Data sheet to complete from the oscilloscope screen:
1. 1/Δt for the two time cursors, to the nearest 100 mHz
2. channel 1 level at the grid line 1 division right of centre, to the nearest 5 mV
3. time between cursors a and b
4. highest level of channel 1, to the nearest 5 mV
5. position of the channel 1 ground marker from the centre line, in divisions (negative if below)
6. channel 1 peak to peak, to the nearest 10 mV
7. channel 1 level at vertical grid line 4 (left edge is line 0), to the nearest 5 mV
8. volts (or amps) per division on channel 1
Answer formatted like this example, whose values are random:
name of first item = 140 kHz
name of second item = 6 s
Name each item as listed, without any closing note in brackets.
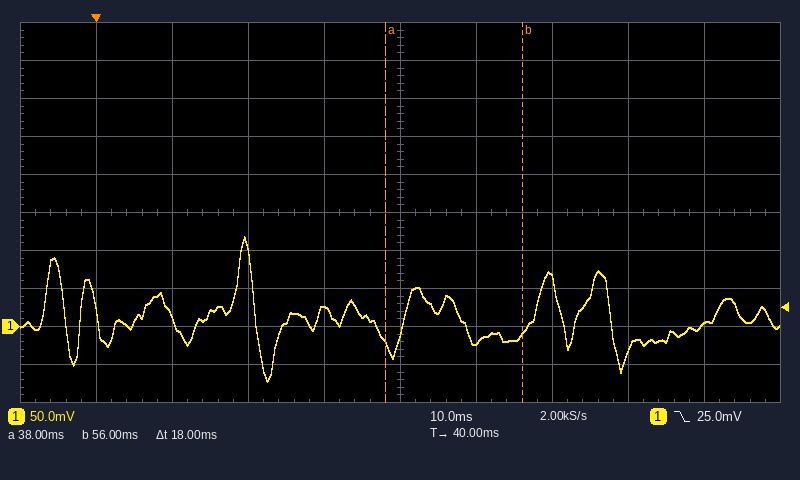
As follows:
1/Δt for the two time cursors, to the nearest 100 mHz = 55.6 Hz
channel 1 level at the grid line 1 division right of centre, to the nearest 5 mV = -20 mV
time between cursors a and b = 18 ms
highest level of channel 1, to the nearest 5 mV = 120 mV
position of the channel 1 ground marker from the centre line, in divisions = -3.0 div
channel 1 peak to peak, to the nearest 10 mV = 190 mV
channel 1 level at vertical grid line 4 (left edge is line 0), to the nearest 5 mV = 25 mV
volts (or amps) per division on channel 1 = 50 mV
